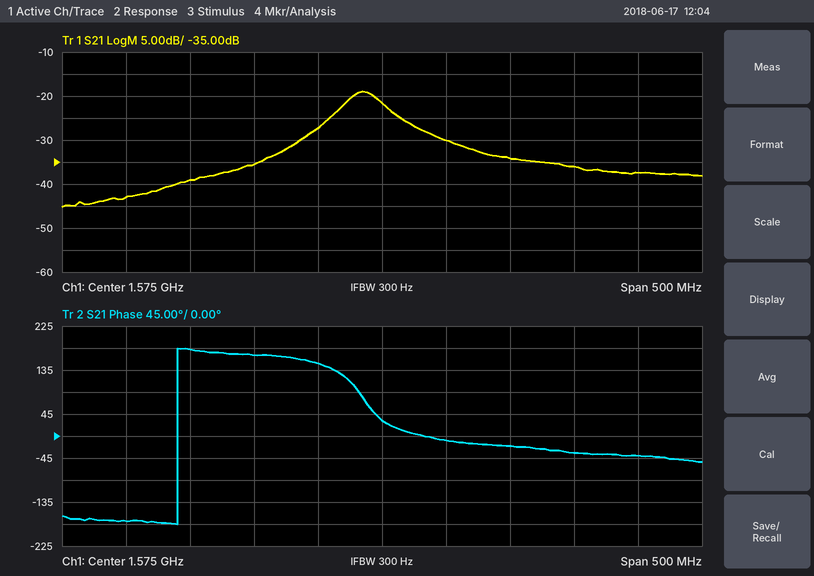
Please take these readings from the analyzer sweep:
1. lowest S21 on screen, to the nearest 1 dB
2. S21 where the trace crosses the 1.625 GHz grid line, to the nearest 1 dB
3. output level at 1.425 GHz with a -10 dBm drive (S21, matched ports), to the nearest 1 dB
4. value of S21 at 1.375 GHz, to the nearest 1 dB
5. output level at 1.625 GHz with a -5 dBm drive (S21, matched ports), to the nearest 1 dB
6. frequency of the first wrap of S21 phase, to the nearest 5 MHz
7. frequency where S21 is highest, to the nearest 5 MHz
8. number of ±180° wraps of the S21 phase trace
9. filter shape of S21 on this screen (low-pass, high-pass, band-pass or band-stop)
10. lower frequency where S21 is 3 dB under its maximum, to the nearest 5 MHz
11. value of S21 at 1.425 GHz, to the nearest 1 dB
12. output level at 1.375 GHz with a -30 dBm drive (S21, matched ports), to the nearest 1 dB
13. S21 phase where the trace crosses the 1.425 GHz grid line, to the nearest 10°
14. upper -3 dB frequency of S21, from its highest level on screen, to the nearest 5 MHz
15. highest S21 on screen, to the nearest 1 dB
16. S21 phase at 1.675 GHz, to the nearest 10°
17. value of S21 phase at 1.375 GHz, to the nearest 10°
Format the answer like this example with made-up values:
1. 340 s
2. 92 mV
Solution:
1. -45 dB
2. -30 dB
3. -49 dBm
4. -43 dB
5. -35 dBm
6. 1.415 GHz
7. 1.560 GHz
8. 1
9. band-pass
10. 1.545 GHz
11. -39 dB
12. -73 dBm
13. 180°
14. 1.575 GHz
15. -19 dB
16. -20°
17. -170°
